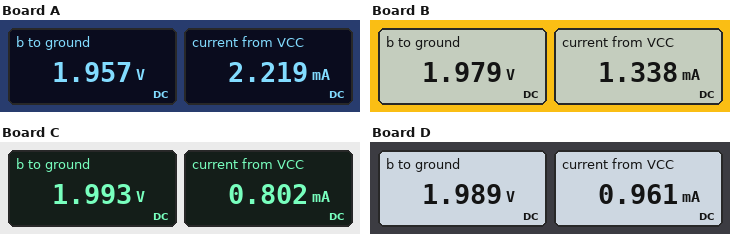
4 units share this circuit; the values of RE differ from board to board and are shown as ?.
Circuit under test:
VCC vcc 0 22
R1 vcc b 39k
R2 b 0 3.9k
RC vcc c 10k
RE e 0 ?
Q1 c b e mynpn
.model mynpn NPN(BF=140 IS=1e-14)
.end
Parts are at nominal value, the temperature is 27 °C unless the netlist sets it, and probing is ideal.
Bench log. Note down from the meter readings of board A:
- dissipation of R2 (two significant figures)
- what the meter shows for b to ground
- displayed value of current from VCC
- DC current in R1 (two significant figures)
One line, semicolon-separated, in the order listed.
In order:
980 µW; 1.957 V; 2.219 mA; 510 µA
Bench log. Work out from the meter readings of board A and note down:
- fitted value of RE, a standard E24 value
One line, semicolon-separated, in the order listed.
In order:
750 Ω
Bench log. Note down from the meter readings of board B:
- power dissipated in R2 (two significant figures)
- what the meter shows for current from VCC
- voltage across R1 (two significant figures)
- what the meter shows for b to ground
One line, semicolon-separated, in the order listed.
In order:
1.0 mW; 1.338 mA; 20 V; 1.979 V
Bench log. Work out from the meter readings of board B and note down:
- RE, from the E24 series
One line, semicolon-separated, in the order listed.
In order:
1.6 kΩ
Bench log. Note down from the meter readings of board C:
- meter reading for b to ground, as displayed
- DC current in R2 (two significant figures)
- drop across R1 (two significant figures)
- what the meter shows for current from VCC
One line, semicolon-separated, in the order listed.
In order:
1.993 V; 510 µA; 20 V; 0.802 mA
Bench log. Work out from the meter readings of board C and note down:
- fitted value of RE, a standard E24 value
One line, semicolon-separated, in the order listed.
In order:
4.7 kΩ
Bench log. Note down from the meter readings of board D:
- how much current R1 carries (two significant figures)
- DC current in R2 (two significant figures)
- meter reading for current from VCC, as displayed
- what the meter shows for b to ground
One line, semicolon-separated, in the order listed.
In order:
510 µA; 510 µA; 0.961 mA; 1.989 V
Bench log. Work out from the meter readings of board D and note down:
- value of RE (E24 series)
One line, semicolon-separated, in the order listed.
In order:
3 kΩ
